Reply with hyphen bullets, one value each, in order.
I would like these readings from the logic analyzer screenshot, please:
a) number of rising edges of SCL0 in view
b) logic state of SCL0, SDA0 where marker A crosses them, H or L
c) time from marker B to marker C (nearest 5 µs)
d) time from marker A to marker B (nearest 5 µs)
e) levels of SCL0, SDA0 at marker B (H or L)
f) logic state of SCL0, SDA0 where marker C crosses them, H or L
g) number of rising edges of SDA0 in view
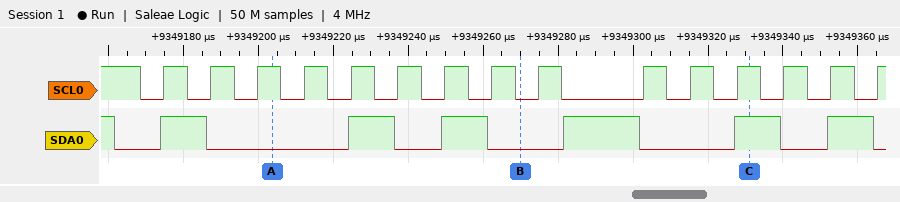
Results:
- 15
- SCL0=H, SDA0=L
- 60 µs
- 65 µs
- SCL0=L, SDA0=L
- SCL0=H, SDA0=H
- 6
